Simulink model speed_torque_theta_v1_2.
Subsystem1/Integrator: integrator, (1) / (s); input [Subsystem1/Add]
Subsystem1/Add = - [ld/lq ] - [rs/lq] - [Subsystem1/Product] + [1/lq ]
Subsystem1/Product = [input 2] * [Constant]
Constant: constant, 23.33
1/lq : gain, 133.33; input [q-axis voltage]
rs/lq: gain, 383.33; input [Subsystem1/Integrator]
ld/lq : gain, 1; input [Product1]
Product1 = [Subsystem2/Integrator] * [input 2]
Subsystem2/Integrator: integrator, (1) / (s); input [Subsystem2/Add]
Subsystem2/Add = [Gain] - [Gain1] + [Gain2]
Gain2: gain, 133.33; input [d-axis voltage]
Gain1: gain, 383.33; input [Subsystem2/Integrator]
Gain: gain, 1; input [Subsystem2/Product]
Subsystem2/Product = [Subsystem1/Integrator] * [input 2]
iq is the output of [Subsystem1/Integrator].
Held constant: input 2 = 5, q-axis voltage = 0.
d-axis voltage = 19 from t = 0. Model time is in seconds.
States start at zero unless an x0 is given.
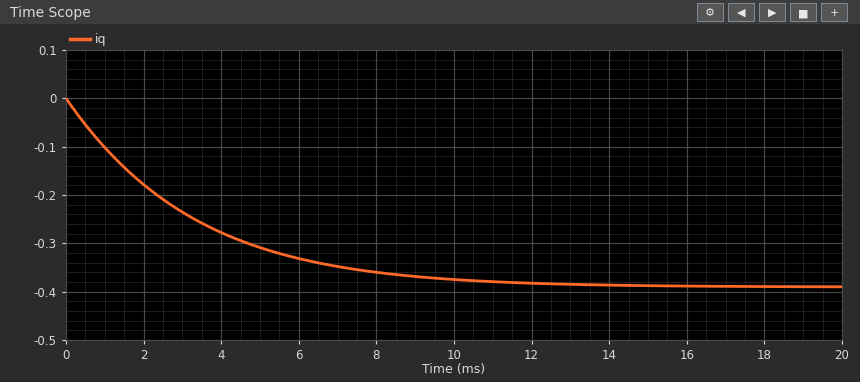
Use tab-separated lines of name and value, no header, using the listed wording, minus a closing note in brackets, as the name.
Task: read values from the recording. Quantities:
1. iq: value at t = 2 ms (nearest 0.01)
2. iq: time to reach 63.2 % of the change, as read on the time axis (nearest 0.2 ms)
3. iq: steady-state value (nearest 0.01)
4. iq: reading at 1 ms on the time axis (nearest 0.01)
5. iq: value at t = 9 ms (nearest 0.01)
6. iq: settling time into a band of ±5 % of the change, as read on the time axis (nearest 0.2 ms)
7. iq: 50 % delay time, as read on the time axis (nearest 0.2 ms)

iq: value at t = 2 ms	-0.18
iq: time to reach 63.2 % of the change, as read on the time axis	3.2 ms
iq: steady-state value	-0.39
iq: reading at 1 ms on the time axis	-0.10
iq: value at t = 9 ms	-0.37
iq: settling time into a band of ±5 % of the change, as read on the time axis	9.4 ms
iq: 50 % delay time, as read on the time axis	2.2 ms
